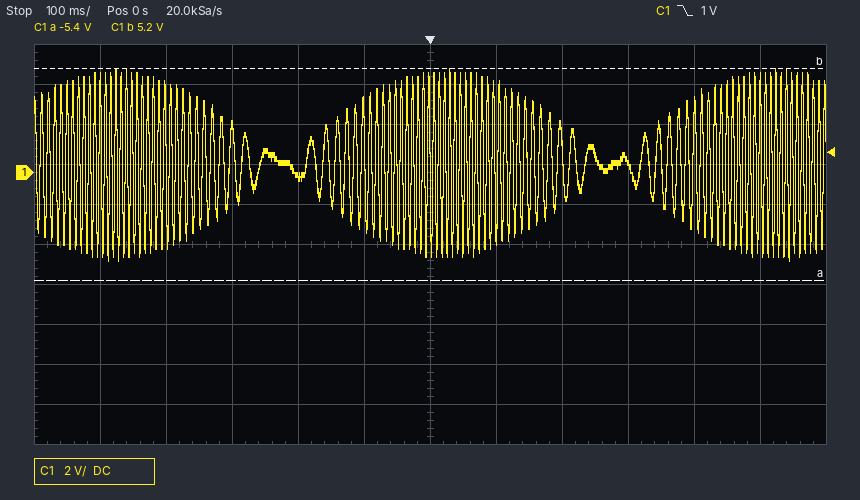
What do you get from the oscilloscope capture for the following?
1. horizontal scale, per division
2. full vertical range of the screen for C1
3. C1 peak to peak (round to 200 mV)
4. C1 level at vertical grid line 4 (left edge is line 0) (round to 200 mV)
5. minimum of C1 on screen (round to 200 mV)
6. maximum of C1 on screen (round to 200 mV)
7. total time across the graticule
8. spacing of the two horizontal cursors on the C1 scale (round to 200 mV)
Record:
100 ms
20 V
9.6 V
-200 mV
-4.4 V
5.2 V
1.2 s
10.6 V
